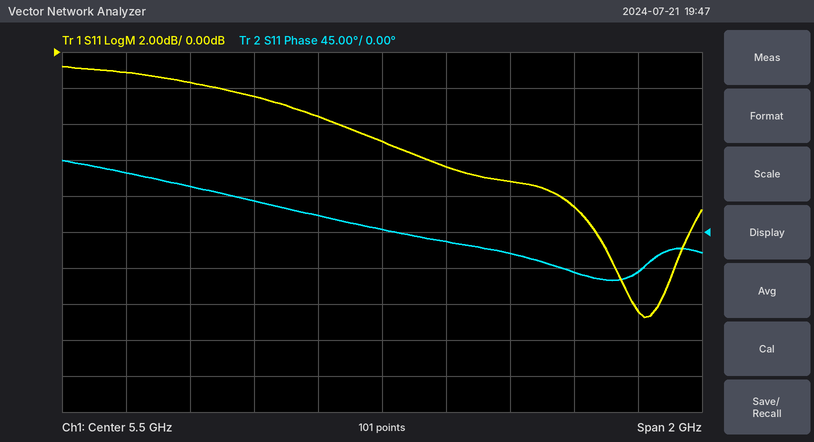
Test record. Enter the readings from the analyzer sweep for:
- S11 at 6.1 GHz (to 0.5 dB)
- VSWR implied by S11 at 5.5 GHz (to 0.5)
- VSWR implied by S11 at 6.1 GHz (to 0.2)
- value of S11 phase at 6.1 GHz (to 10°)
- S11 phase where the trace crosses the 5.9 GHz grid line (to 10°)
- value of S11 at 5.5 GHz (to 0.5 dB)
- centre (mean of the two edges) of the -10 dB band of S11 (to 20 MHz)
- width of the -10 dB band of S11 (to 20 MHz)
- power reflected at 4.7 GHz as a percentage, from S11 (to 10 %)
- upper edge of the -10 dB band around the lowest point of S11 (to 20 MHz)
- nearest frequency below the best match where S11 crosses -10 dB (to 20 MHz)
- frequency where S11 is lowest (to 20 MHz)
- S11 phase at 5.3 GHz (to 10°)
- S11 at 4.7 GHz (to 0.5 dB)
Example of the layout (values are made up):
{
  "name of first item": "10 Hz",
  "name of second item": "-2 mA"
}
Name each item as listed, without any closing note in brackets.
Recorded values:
{
  "S11 at 6.1 GHz": "-8.5 dB",
  "VSWR implied by S11 at 5.5 GHz": "3.5",
  "VSWR implied by S11 at 6.1 GHz": "2.2",
  "value of S11 phase at 6.1 GHz": "-50°",
  "S11 phase where the trace crosses the 5.9 GHz grid line": "-30°",
  "value of S11 at 5.5 GHz": "-5.0 dB",
  "centre (mean of the two edges) of the -10 dB band of S11": "6.32 GHz",
  "width of the -10 dB band of S11": "300 MHz",
  "power reflected at 4.7 GHz as a percentage, from S11": "80 %",
  "upper edge of the -10 dB band around the lowest point of S11": "6.46 GHz",
  "nearest frequency below the best match where S11 crosses -10 dB": "6.16 GHz",
  "frequency where S11 is lowest": "6.32 GHz",
  "S11 phase at 5.3 GHz": "20°",
  "S11 at 4.7 GHz": "-1.0 dB"
}
